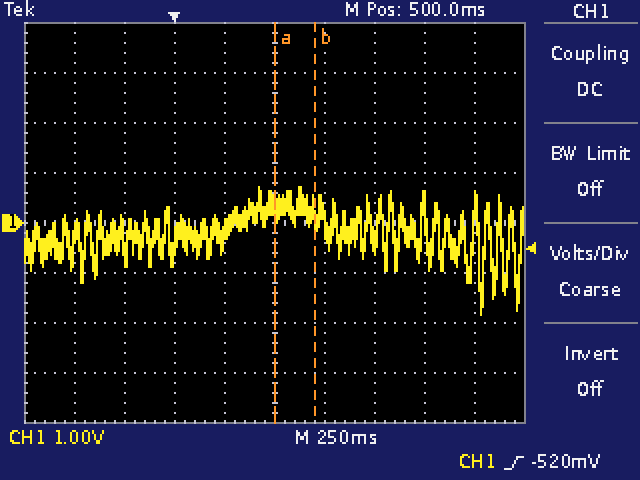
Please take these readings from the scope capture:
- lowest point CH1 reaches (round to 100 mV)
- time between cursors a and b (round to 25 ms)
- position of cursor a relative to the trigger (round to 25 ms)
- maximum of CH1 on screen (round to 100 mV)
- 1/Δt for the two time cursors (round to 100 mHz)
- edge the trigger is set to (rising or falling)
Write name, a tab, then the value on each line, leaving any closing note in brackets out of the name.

lowest point CH1 reaches	-1.8 V
time between cursors a and b	200 ms
position of cursor a relative to the trigger	+500 ms
maximum of CH1 on screen	700 mV
1/Δt for the two time cursors	5.0 Hz
edge the trigger is set to	rising
